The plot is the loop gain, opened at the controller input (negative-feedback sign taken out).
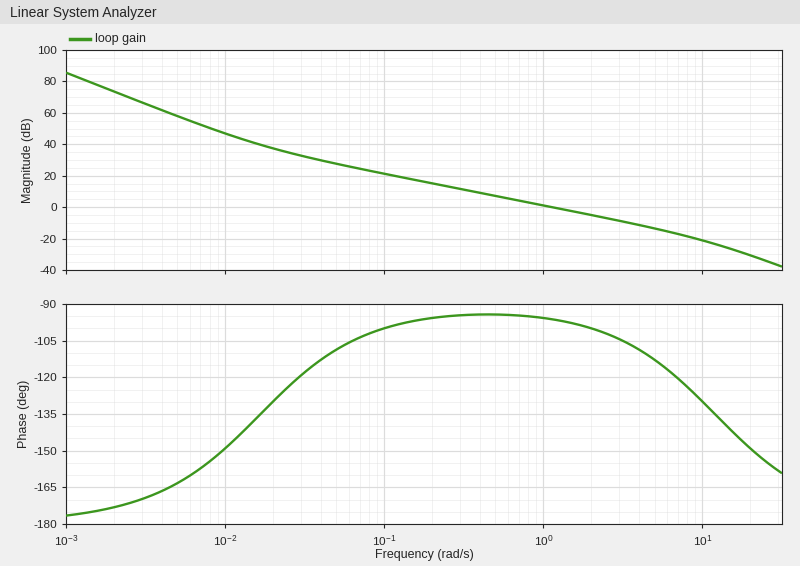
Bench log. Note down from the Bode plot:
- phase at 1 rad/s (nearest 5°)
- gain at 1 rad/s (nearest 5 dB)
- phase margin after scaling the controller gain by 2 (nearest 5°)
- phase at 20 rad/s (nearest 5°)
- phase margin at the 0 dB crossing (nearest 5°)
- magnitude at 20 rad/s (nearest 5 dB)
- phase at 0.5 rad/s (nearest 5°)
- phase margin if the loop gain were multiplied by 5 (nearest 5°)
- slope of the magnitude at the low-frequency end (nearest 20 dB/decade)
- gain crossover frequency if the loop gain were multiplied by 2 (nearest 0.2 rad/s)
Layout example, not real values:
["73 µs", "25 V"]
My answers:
["-95°", "0 dB", "80°", "-150°", "85°", "-30 dB", "-95°", "65°", "-40 dB/decade", "2.2 rad/s"]
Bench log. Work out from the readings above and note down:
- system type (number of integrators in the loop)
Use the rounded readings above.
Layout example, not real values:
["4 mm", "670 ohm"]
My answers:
["2"]
